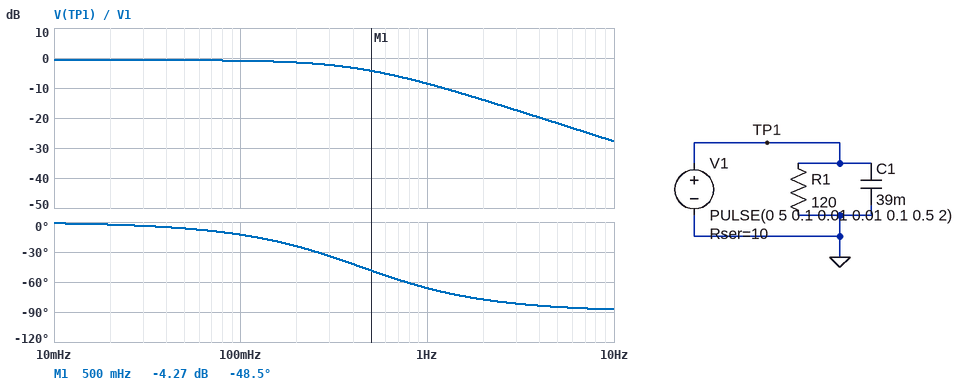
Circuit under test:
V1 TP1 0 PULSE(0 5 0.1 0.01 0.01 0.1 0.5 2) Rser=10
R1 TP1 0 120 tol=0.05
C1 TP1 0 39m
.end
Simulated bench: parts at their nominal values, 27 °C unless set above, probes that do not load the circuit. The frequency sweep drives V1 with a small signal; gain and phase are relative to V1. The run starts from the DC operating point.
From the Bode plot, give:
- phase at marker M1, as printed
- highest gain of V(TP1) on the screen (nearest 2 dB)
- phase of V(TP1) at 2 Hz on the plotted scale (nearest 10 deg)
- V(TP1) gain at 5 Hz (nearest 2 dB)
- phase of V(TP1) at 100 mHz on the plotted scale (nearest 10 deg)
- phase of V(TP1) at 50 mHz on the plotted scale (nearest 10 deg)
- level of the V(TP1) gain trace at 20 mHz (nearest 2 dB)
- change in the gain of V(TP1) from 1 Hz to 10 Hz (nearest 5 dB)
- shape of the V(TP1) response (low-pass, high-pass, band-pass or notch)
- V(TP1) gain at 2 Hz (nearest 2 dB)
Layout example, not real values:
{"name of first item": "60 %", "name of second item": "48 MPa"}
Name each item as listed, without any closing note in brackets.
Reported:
{"phase at marker M1, as printed": "-48.5 deg", "highest gain of V(TP1) on the screen": "0 dB", "phase of V(TP1) at 2 Hz on the plotted scale": "-80 deg", "V(TP1) gain at 5 Hz": "-22 dB", "phase of V(TP1) at 100 mHz on the plotted scale": "-10 deg", "phase of V(TP1) at 50 mHz on the plotted scale": "-10 deg", "level of the V(TP1) gain trace at 20 mHz": "0 dB", "change in the gain of V(TP1) from 1 Hz to 10 Hz": "-20 dB", "shape of the V(TP1) response": "low-pass", "V(TP1) gain at 2 Hz": "-14 dB"}
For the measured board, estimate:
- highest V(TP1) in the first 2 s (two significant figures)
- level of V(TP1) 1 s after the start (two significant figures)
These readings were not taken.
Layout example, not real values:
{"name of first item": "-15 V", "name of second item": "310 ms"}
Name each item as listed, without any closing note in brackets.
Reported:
{"highest V(TP1) in the first 2 s": "1.5 V", "level of V(TP1) 1 s after the start": "690 mV"}
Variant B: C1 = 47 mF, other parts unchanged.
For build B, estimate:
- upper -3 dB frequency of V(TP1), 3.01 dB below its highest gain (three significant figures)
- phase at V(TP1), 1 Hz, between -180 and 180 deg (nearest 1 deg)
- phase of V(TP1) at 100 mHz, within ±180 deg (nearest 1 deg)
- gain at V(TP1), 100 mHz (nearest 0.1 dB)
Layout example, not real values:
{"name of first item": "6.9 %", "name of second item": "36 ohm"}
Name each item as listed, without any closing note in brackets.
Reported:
{"upper -3 dB frequency of V(TP1), 3.01 dB below its highest gain": "367 mHz", "phase at V(TP1), 1 Hz, between -180 and 180 deg": "-70 deg", "phase of V(TP1) at 100 mHz, within ±180 deg": "-15 deg", "gain at V(TP1), 100 mHz": "-1.0 dB"}
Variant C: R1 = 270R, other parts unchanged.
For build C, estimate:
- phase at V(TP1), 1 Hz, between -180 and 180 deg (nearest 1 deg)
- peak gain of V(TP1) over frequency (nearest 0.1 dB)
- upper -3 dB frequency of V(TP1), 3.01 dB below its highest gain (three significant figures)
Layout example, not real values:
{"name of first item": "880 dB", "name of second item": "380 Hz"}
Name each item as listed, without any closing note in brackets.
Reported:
{"phase at V(TP1), 1 Hz, between -180 and 180 deg": "-67 deg", "peak gain of V(TP1) over frequency": "-0.3 dB", "upper -3 dB frequency of V(TP1), 3.01 dB below its highest gain": "423 mHz"}
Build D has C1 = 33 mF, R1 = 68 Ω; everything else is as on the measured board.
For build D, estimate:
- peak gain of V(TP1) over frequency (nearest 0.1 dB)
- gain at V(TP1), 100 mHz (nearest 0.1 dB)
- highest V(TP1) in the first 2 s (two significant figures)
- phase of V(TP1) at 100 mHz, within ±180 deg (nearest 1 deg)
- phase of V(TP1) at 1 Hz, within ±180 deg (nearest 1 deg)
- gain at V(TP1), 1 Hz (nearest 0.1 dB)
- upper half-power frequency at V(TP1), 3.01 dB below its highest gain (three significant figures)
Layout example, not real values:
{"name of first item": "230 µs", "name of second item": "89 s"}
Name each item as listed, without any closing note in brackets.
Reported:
{"peak gain of V(TP1) over frequency": "-1.2 dB", "gain at V(TP1), 100 mHz": "-1.3 dB", "highest V(TP1) in the first 2 s": "1.6 V", "phase of V(TP1) at 100 mHz, within ±180 deg": "-10 deg", "phase of V(TP1) at 1 Hz, within ±180 deg": "-61 deg", "gain at V(TP1), 1 Hz": "-7.5 dB", "upper half-power frequency at V(TP1), 3.01 dB below its highest gain": "553 mHz"}
